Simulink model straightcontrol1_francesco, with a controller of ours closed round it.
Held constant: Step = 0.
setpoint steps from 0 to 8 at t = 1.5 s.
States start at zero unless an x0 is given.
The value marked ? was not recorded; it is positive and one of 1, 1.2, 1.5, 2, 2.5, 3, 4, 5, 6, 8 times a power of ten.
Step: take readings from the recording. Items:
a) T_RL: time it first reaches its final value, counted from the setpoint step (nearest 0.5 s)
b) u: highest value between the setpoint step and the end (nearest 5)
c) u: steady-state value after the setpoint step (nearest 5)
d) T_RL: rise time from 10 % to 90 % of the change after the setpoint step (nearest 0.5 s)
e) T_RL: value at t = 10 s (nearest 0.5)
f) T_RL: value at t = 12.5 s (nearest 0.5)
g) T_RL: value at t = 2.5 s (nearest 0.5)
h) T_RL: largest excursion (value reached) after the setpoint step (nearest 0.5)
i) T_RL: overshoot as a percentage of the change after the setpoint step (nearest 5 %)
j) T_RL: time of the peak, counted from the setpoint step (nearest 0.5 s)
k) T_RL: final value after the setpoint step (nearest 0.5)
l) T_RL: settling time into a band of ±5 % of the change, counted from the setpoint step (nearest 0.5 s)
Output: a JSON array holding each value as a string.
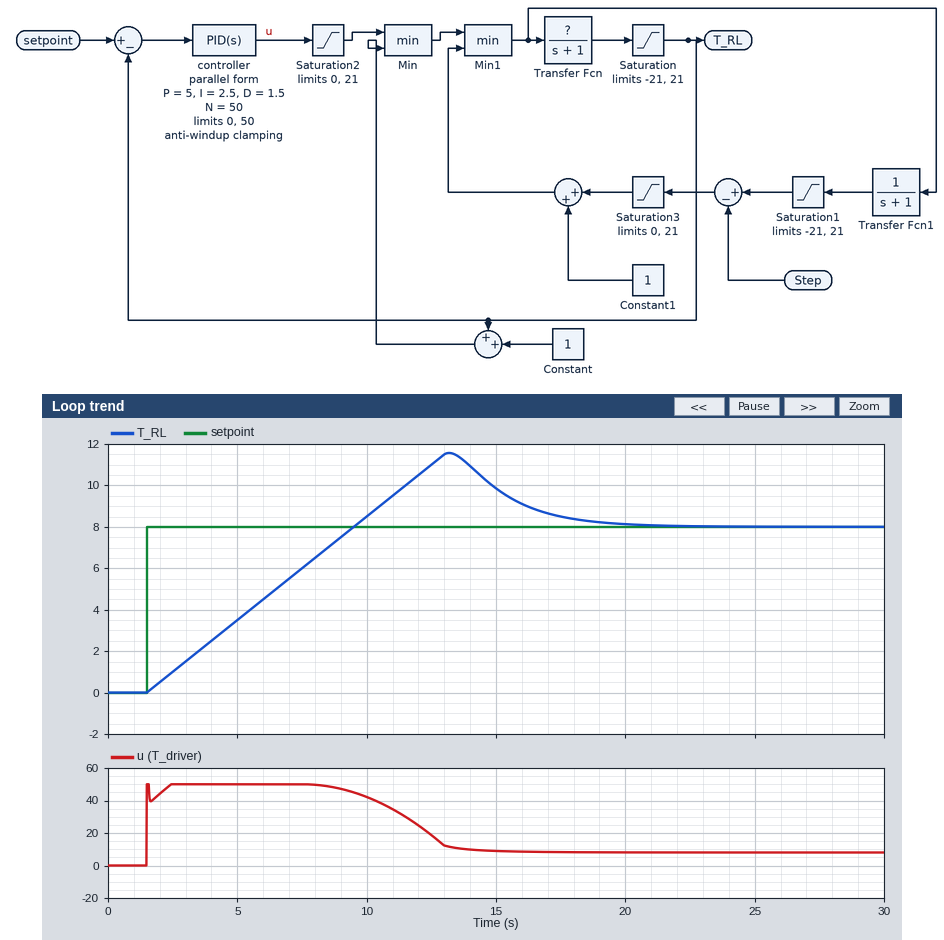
["8.0 s", "50", "10", "6.5 s", "8.5", "11.0", "1.0", "11.5", "45 %", "11.5 s", "8.0", "16.5 s"]
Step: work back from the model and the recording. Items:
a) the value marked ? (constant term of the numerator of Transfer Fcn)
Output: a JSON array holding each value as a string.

["1"]
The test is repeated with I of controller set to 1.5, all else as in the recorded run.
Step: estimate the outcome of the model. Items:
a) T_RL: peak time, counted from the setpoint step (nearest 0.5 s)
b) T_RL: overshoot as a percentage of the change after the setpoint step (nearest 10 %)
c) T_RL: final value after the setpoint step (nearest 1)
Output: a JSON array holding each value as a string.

["12.0 s", "50 %", "8"]
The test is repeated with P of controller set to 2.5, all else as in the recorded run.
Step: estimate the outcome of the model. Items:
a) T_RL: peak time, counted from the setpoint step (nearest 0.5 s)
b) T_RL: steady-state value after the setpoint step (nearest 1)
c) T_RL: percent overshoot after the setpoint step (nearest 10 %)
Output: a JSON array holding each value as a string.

["12.5 s", "8", "60 %"]
